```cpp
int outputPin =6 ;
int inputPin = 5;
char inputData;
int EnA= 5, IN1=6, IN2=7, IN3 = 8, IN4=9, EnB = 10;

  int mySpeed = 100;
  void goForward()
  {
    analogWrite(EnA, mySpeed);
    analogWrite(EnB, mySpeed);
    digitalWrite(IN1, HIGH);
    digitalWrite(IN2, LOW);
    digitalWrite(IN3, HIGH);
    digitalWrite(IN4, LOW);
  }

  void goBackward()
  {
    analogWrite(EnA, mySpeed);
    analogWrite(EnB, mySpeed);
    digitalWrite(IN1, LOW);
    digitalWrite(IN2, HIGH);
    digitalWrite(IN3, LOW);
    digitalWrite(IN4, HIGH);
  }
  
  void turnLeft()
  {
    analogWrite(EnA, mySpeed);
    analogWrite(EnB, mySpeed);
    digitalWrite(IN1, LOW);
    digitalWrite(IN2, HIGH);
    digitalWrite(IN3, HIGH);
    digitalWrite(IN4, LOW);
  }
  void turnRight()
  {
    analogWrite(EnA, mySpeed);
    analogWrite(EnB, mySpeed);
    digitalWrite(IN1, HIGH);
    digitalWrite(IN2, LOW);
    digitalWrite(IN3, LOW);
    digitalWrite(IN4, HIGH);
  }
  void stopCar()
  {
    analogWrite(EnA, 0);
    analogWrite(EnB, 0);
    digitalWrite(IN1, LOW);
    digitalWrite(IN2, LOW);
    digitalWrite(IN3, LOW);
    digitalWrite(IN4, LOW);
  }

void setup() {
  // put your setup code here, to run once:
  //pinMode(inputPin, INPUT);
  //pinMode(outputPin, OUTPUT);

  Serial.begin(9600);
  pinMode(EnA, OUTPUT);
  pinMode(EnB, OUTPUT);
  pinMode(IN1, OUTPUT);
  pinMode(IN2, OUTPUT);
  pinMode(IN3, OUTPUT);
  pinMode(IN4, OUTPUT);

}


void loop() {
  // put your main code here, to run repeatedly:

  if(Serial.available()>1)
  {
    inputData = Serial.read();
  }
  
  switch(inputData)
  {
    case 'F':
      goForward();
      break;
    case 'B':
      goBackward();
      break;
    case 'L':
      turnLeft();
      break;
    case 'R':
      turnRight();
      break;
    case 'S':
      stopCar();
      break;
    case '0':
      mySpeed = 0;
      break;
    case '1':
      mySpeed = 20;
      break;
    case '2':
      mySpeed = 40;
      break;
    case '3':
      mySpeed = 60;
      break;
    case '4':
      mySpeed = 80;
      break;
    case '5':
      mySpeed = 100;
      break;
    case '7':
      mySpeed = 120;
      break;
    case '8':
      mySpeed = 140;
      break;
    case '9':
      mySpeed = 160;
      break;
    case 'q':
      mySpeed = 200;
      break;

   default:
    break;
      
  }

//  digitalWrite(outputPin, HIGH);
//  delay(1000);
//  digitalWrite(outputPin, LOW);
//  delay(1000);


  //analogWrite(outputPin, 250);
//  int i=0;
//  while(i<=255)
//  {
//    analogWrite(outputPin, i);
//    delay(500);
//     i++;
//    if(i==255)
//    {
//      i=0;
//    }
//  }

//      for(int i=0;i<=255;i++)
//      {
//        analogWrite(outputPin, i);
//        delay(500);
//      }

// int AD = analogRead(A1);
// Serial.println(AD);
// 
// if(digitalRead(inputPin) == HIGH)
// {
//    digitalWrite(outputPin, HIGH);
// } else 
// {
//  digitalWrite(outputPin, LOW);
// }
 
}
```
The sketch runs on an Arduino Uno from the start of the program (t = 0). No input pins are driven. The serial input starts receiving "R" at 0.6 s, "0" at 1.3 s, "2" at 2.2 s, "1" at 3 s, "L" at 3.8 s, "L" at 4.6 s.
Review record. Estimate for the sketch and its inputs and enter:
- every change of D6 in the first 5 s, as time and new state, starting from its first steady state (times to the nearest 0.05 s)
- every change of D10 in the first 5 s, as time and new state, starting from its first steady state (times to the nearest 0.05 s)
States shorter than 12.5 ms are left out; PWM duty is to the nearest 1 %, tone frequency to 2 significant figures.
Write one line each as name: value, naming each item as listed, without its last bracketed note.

every change of D6 in the first 5 s, as time and new state, starting from its first steady state: 0 s low; 1.3 s high; 4.6 s low
every change of D10 in the first 5 s, as time and new state, starting from its first steady state: 0 s low; 1.3 s PWM 39 %; 4.6 s PWM 8 %
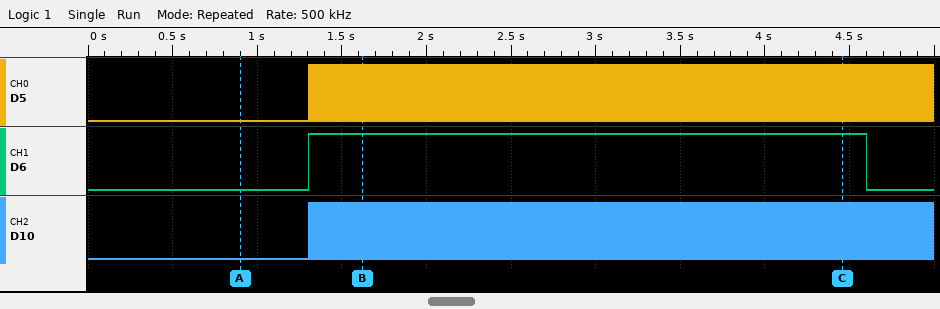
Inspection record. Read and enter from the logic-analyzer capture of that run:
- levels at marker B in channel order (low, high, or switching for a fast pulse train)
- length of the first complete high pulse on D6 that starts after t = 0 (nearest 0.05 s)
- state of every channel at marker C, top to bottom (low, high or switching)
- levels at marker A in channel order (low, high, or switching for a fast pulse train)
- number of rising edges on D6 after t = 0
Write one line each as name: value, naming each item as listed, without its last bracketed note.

levels at marker B in channel order: D5 switching, D6 high, D10 switching
length of the first complete high pulse on D6 that starts after t = 0: 3.30 s
state of every channel at marker C, top to bottom: D5 switching, D6 high, D10 switching
levels at marker A in channel order: D5 low, D6 low, D10 low
number of rising edges on D6 after t = 0: 1
